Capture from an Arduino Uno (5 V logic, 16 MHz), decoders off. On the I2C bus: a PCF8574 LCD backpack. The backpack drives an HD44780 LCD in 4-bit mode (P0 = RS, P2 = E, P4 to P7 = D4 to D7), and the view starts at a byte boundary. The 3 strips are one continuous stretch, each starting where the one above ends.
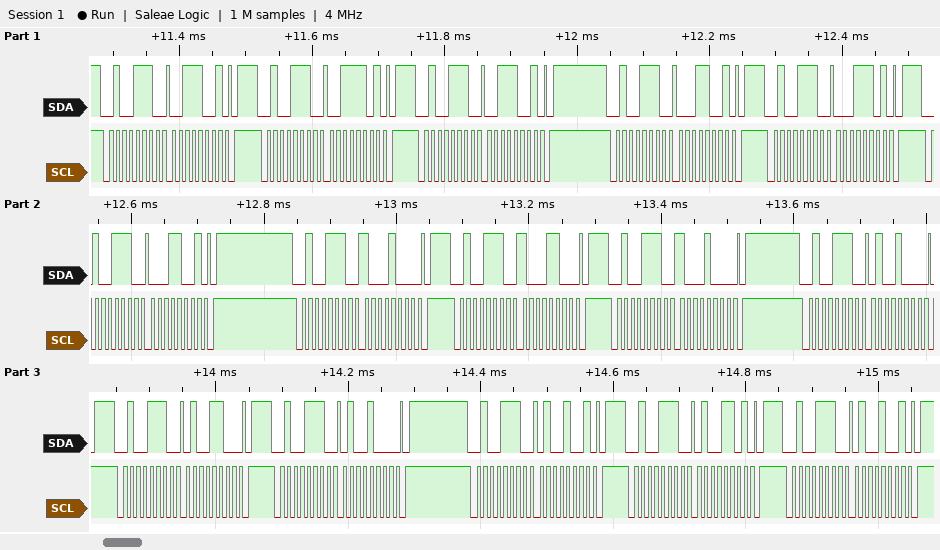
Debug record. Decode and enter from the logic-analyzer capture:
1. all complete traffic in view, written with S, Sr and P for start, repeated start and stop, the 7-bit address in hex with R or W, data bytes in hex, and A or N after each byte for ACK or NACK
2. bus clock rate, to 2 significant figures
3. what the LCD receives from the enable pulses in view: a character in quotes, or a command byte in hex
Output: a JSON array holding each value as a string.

["S 27W A 39 A P S 27W A 3D A P S 27W A 39 A P S 27W A 19 A P S 27W A 1D A P S 27W A 19 A P S 27W A 88 A P S 27W A 8C A P S 27W A 88 A P S 27W A 48 A P S 27W A 4C A P S 27W A 48 A P S 27W A 49 A P S 27W A 4D A P S 27W A 49 A P", "100 kHz", "'1' 0x84"]
